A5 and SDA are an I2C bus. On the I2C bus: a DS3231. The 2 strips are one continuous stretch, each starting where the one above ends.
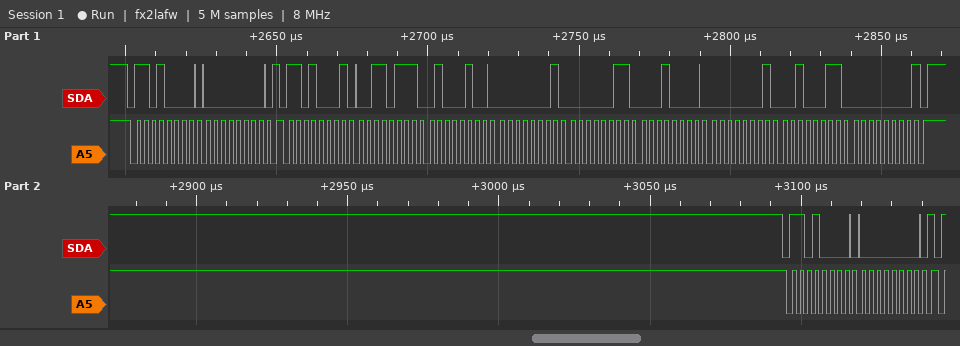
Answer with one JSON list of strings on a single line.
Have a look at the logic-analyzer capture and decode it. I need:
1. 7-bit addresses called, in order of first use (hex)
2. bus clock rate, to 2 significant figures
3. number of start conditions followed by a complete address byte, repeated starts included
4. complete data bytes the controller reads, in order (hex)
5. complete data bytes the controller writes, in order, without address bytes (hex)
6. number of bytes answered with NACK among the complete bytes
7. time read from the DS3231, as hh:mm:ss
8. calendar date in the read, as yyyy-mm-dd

["0x68", "400 kHz", "3", "37 44 01 03 10 01 23 00", "00 00", "1", "01:44:37", "2023-01-10"]
